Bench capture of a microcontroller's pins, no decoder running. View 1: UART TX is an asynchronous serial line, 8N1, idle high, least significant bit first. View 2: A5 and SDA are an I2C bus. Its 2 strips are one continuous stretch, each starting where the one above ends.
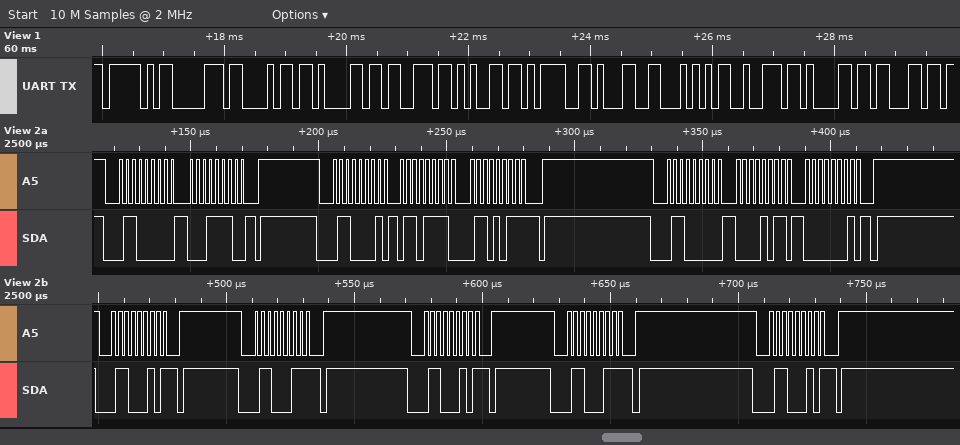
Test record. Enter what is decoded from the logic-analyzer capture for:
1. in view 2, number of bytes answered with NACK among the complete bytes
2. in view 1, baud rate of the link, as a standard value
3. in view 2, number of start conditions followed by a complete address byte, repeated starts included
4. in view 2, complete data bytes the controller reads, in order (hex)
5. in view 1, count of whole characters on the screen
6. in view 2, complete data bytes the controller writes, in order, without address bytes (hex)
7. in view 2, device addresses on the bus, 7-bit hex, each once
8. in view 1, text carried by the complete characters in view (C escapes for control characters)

6
9600 baud
8
6F 6B
12
1E 0B 01
0x30 0x31
"_phase=1Trac"
